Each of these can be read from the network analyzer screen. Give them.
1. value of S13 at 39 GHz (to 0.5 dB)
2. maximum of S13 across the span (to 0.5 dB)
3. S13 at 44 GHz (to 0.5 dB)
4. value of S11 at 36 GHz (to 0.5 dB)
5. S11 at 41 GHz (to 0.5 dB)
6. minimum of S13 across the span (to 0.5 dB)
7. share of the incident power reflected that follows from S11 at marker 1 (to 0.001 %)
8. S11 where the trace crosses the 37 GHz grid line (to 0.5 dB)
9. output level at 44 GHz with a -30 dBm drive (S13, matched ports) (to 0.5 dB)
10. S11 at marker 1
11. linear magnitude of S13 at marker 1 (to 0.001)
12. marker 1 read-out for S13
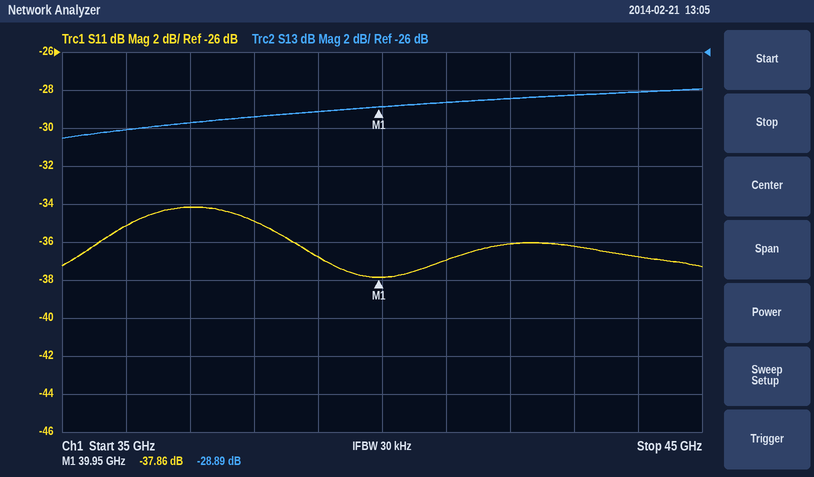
-29.0 dB
-28.0 dB
-28.0 dB
-35.0 dB
-37.0 dB
-30.5 dB
0.016 %
-34.0 dB
-58.0 dBm
-37.86 dB
0.036
-28.89 dB
